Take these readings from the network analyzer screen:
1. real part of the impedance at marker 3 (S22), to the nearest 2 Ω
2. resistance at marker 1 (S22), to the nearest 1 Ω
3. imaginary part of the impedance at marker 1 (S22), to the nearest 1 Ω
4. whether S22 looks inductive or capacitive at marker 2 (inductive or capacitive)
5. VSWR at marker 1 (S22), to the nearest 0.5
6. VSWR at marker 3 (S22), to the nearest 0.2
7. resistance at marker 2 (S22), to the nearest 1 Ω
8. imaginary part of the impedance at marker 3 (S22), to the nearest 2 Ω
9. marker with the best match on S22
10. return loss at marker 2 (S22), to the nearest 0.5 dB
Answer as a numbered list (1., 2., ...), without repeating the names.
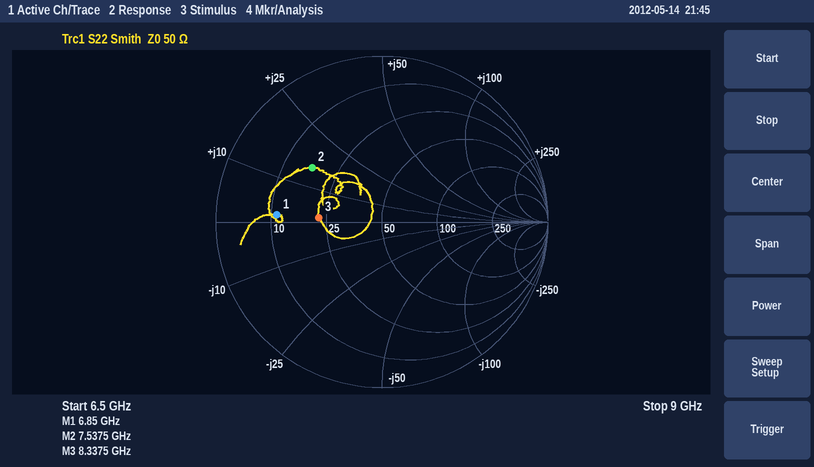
1. 22 Ω
2. 11 Ω
3. +2 Ω
4. inductive
5. 4.5
6. 2.2
7. 17 Ω
8. +2 Ω
9. marker 3
10. 5.5 dB
